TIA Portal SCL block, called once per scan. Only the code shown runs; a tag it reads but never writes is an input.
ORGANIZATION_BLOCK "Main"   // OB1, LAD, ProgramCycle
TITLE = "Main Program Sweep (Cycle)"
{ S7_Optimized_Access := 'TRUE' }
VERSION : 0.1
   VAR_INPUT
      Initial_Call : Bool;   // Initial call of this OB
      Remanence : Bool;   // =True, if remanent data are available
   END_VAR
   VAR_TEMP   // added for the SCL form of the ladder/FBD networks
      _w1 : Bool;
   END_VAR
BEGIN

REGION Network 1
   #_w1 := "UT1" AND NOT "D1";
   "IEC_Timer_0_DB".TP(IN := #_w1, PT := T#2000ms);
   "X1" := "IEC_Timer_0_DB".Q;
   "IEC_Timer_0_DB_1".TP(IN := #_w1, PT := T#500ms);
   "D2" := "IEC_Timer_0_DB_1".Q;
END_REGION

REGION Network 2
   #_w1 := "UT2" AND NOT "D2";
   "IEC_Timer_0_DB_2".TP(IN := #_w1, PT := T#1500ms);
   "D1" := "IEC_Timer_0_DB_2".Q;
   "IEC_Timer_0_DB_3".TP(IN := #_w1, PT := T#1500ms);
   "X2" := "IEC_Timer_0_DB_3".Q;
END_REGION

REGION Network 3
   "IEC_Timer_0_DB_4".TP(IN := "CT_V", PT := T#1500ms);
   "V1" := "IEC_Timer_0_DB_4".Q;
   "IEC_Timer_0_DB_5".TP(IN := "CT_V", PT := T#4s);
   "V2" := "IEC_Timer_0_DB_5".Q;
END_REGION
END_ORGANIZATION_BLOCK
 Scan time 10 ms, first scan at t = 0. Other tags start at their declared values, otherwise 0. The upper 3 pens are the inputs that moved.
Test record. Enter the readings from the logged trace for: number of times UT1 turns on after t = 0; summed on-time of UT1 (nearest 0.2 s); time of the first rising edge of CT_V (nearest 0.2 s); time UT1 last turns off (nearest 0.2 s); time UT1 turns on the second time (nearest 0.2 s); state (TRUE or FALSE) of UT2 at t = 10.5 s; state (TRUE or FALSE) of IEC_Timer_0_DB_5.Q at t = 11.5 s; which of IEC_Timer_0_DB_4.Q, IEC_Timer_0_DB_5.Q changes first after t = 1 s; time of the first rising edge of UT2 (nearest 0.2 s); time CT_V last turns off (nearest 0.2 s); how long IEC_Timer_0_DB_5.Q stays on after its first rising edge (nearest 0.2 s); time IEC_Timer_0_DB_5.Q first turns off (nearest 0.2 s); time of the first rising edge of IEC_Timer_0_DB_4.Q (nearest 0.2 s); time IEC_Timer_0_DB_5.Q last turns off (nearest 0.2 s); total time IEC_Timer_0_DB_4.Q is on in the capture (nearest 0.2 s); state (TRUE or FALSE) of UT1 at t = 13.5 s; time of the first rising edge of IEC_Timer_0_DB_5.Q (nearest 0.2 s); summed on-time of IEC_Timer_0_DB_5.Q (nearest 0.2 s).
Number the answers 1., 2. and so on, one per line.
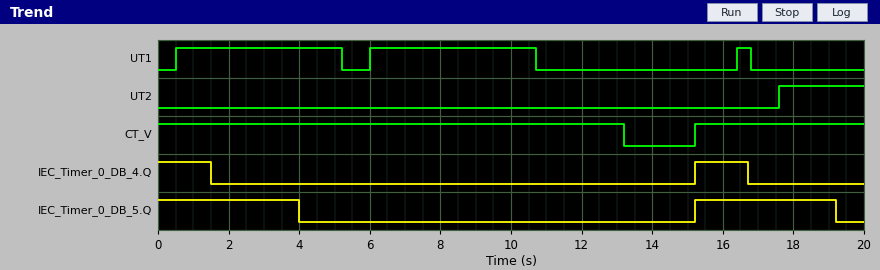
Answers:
1. 3
2. 9.8 s
3. 15.2 s
4. 16.8 s
5. 6.0 s
6. FALSE
7. FALSE
8. IEC_Timer_0_DB_4.Q
9. 17.6 s
10. 13.2 s
11. 4.0 s
12. 4.0 s
13. 15.2 s
14. 19.2 s
15. 3.0 s
16. FALSE
17. 15.2 s
18. 8.0 s
